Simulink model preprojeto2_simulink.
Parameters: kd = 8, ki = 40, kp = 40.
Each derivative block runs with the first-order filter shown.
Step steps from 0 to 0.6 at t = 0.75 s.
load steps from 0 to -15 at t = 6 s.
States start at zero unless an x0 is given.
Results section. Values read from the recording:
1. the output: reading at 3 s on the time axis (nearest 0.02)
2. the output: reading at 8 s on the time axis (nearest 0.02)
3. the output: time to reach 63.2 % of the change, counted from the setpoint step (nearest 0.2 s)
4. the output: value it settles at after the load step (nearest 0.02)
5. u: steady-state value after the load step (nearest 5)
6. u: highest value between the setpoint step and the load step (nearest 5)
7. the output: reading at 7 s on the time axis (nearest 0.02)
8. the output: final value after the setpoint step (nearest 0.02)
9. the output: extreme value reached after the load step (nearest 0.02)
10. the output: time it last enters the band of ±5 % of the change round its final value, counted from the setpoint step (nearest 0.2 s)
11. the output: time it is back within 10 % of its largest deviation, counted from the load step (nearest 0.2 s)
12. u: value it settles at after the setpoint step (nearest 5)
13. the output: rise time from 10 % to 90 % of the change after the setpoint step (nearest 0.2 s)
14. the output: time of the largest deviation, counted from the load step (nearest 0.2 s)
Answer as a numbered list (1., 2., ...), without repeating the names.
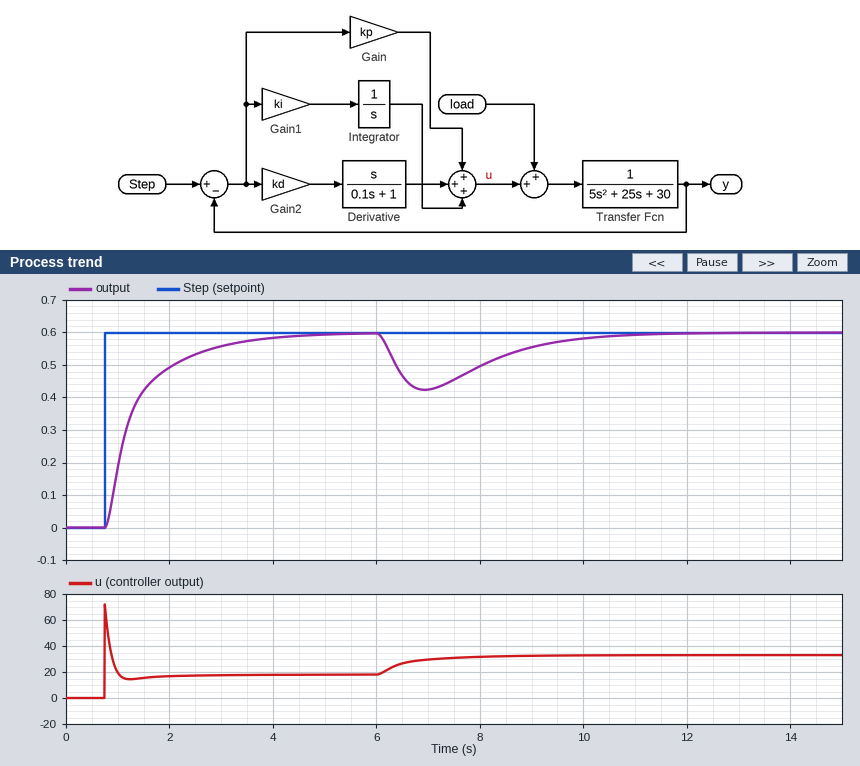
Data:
1. 0.56
2. 0.50
3. 0.6 s
4. 0.60
5. 35
6. 70
7. 0.42
8. 0.60
9. 0.42
10. 2.6 s
11. 4.0 s
12. 20
13. 1.8 s
14. 1.0 s
